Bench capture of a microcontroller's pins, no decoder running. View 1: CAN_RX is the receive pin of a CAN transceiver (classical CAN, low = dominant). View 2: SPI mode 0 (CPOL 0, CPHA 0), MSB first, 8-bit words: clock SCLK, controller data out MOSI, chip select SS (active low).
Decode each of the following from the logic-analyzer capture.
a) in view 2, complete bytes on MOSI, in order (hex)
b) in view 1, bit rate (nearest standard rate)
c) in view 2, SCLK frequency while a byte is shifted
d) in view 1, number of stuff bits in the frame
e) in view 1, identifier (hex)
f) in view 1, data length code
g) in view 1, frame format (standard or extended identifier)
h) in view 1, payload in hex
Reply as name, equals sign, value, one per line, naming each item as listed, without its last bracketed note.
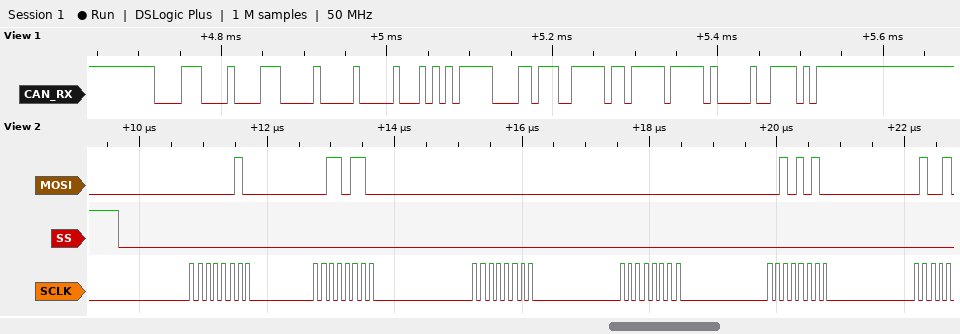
in view 2, complete bytes on MOSI, in order = 02 36 00 00 2A
in view 1, bit rate = 125 kbit/s
in view 2, SCLK frequency while a byte is shifted = 8 MHz
in view 1, number of stuff bits in the frame = 8
in view 1, identifier = 0x0E1
in view 1, data length code = 7
in view 1, frame format = standard
in view 1, payload in hex = 00 00 2A F8 DC FE FF
